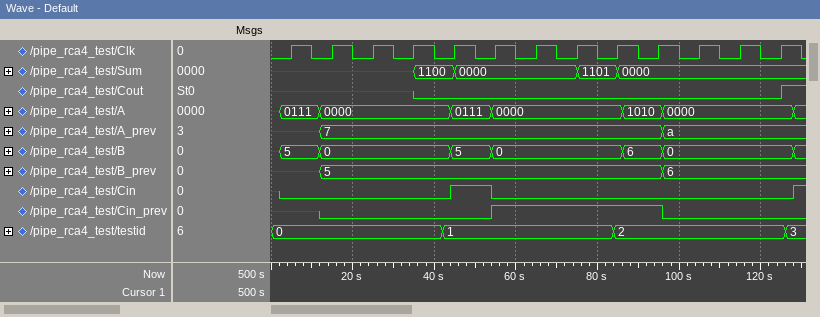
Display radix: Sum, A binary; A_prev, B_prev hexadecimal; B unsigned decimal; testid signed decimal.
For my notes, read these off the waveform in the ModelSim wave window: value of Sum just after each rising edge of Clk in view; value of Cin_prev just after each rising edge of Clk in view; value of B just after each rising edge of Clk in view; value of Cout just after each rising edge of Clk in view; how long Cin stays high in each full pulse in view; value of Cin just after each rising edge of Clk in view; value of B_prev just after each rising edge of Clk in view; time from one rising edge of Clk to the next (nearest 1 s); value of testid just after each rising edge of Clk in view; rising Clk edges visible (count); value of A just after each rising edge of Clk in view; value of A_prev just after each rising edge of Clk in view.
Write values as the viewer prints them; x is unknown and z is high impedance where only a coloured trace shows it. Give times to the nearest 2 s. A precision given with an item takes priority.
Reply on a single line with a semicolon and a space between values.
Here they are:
x, x, x, 1100, 0000, 0000, 0000, 1101, 0000, 0000, 0000, 0000, 0000; x 0 0 0 0 1 1 1 1 1 0 0 0; 5, 0, 0, 0, 5, 0, 0, 0, 0, 6, 0, 0, 0; x x x 0 0 0 0 0 0 0 0 0 1; 10 s; 0 0 0 0 1 0 0 0 0 0 0 0 0; x, 5, 5, 5, 5, 5, 5, 5, 5, 5, 6, 6, 6; 10 s; 0, 0, 0, 0, 1, 1, 1, 1, 2, 2, 2, 2, 2; 13; 0111, 0000, 0000, 0000, 0111, 0000, 0000, 0000, 0000, 1010, 0000, 0000, 0000; x, 7, 7, 7, 7, 7, 7, 7, 7, 7, a, a, a
